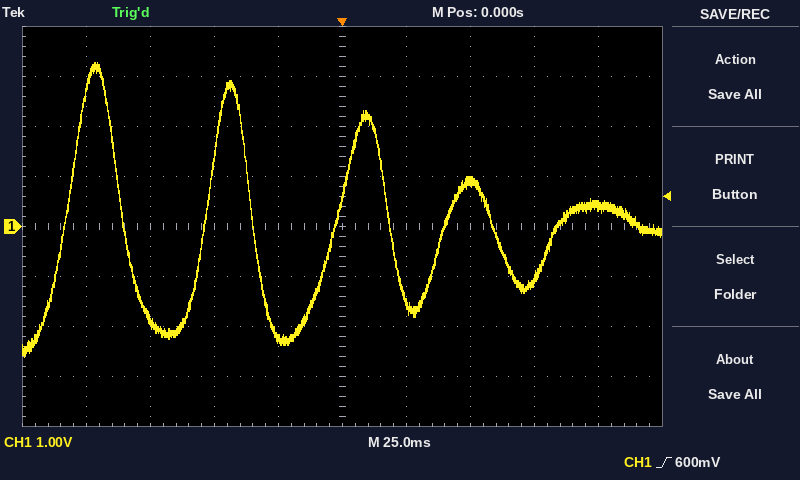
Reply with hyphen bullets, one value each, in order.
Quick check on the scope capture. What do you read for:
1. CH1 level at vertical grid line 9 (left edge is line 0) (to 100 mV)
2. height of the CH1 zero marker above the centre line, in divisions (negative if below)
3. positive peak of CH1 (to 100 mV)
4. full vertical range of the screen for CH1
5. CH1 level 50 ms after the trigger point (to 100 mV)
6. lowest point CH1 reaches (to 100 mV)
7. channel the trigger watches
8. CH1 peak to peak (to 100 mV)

- 400 mV
- 0.0 div
- 3.3 V
- 8 V
- 900 mV
- -2.6 V
- CH1
- 5.9 V
